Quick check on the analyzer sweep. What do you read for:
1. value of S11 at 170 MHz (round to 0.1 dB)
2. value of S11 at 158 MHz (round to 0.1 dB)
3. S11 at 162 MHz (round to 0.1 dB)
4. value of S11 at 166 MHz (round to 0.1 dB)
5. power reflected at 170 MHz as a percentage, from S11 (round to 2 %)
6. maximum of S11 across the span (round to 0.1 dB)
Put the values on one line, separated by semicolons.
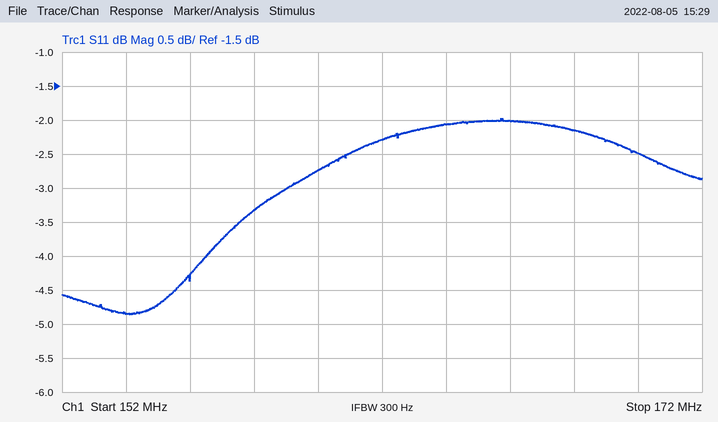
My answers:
-2.5 dB; -3.3 dB; -2.3 dB; -2.0 dB; 56 %; -2.0 dB
